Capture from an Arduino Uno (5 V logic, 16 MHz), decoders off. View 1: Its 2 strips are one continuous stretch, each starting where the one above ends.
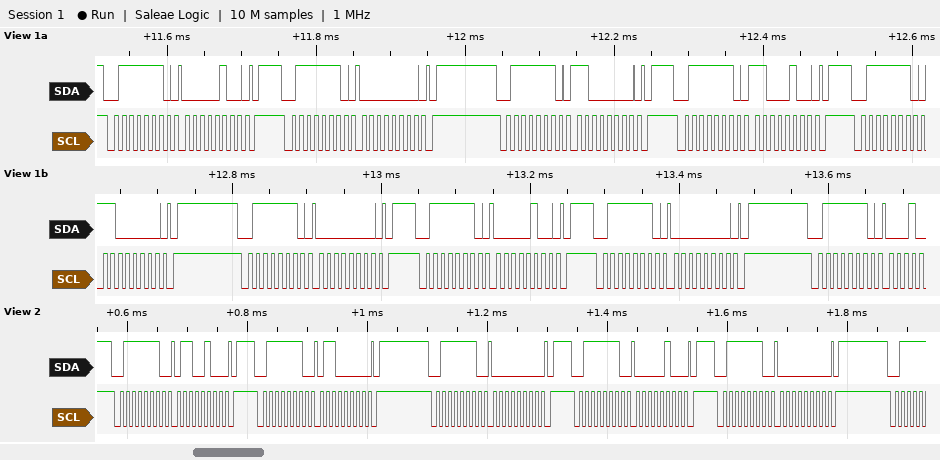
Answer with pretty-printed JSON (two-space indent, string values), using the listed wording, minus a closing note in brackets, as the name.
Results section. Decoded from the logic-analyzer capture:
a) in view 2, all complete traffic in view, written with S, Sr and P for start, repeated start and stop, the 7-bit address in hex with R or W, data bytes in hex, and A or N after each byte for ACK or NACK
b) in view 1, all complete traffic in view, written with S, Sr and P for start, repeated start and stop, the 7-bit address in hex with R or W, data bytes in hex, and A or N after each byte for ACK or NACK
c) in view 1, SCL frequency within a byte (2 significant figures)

{
  "in view 2, all complete traffic in view, written with S, Sr and P for start, repeated start and stop, the 7-bit address in hex with R or W, data bytes in hex, and A or N after each byte for ACK or NACK": "S 3FW A 64 A P S 3FW A 60 A P S 3FW A 00 A P S 3FW A 04 A P S 3FW A 00 A P",
  "in view 1, all complete traffic in view, written with S, Sr and P for start, repeated start and stop, the 7-bit address in hex with R or W, data bytes in hex, and A or N after each byte for ACK or NACK": "S 3FW A 04 A P S 3FW A 00 A P S 3FW A C0 A P S 3FW A C4 A P S 3FW A C0 A P S 3FW A 00 A P S 3FW A 04 A P S 3FW A 00 A P S 3FW A",
  "in view 1, SCL frequency within a byte": "100 kHz"
}
